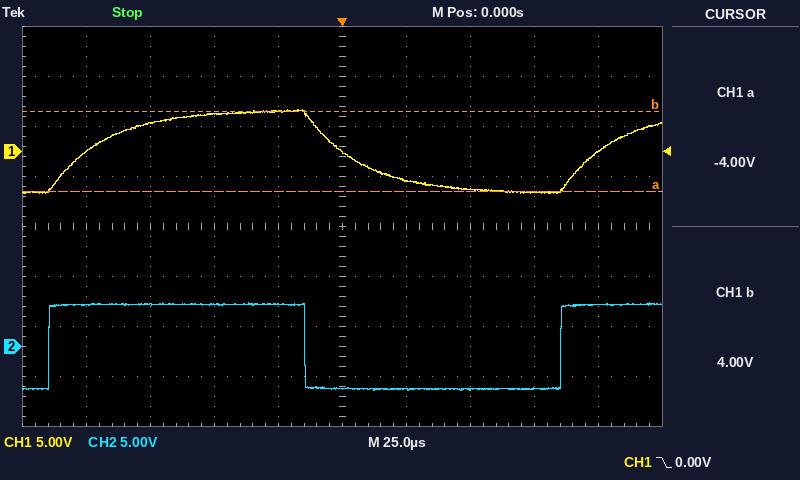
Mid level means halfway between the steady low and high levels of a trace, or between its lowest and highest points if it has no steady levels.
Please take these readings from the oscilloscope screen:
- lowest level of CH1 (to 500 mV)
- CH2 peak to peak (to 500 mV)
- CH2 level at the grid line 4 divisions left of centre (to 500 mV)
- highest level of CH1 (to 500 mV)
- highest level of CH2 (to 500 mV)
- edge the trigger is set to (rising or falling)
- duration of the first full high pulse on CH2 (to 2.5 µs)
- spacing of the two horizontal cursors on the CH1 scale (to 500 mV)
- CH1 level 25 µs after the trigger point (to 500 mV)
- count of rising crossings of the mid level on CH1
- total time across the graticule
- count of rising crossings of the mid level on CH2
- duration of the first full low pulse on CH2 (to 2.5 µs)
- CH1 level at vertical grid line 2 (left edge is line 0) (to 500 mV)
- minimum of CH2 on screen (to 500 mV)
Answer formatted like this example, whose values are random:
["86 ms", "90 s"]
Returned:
["-4.0 V", "9.0 V", "4.0 V", "4.0 V", "4.5 V", "falling", "100.0 µs", "8.0 V", "-3.0 V", "2", "250 µs", "2", "100.0 µs", "3.0 V", "-4.5 V"]
